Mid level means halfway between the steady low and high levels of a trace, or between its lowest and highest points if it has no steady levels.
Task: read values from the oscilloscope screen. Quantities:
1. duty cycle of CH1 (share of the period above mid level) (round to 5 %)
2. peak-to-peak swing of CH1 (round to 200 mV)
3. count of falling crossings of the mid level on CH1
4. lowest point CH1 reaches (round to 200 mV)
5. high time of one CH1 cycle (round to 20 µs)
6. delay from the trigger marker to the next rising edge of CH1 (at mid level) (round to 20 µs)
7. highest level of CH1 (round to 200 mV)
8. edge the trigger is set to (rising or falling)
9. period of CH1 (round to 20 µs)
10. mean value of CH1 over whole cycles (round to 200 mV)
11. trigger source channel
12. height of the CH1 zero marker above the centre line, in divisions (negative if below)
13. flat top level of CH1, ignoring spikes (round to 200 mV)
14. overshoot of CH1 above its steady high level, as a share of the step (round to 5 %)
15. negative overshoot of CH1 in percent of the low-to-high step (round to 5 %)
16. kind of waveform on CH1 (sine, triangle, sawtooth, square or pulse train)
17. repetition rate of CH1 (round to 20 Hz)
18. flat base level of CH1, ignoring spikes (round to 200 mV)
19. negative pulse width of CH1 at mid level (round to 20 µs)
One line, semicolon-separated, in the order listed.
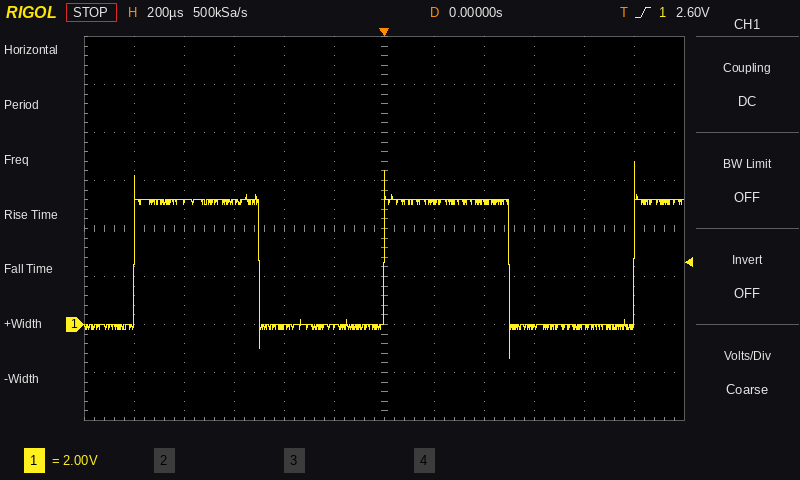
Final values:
50 %; 8.2 V; 2; -1.4 V; 500 µs; 1.00 ms; 6.8 V; rising; 1.00 ms; 2.6 V; CH1; -2.0 div; 5.2 V; 30 %; 25 %; square; 1.00 kHz; 0.0 V; 500 µs
